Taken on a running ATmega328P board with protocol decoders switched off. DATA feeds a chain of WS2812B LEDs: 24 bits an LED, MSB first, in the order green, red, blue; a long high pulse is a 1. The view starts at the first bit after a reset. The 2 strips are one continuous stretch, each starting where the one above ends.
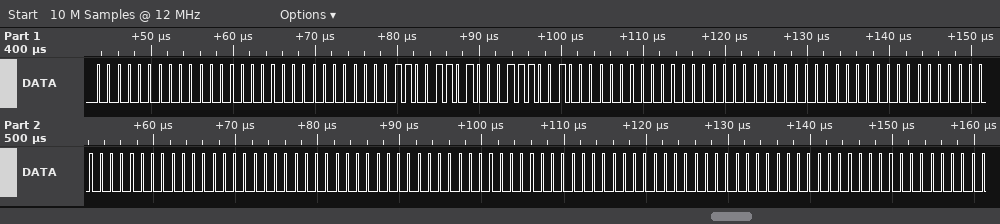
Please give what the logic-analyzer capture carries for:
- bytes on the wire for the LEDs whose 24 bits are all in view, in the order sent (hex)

00 00 00 06 68 E4 00 00 00 00 00 00 00 00 00 00 00 00 00 00 00
